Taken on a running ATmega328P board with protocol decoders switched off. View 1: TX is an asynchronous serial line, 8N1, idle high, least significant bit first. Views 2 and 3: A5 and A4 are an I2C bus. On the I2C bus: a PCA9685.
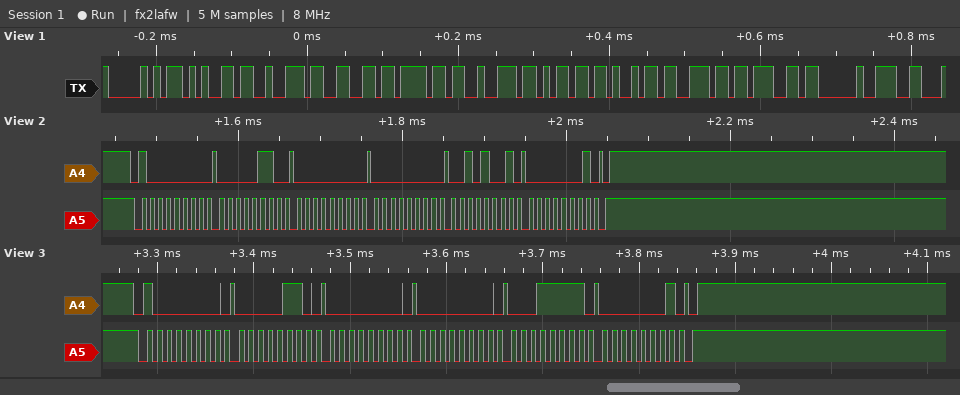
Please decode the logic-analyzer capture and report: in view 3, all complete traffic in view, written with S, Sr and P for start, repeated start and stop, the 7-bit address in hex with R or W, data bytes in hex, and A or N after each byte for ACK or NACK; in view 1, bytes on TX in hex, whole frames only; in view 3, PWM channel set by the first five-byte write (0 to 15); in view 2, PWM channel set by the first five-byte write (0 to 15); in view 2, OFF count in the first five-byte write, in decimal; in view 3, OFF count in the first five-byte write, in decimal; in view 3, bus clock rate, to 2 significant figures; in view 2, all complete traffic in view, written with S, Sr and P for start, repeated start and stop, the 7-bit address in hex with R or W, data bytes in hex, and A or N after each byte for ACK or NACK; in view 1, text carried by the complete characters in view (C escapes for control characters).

S 40W A 06 A 00 A 00 A 1F A 01 A P
0x50 0x65 0x72 0x66 0x6F 0x72 0x6D 0x69 0x6E 0x67 0x20
0
0
297
287
100 kHz
S 40W A 06 A 00 A 00 A 29 A 01 A P
"Performing "
